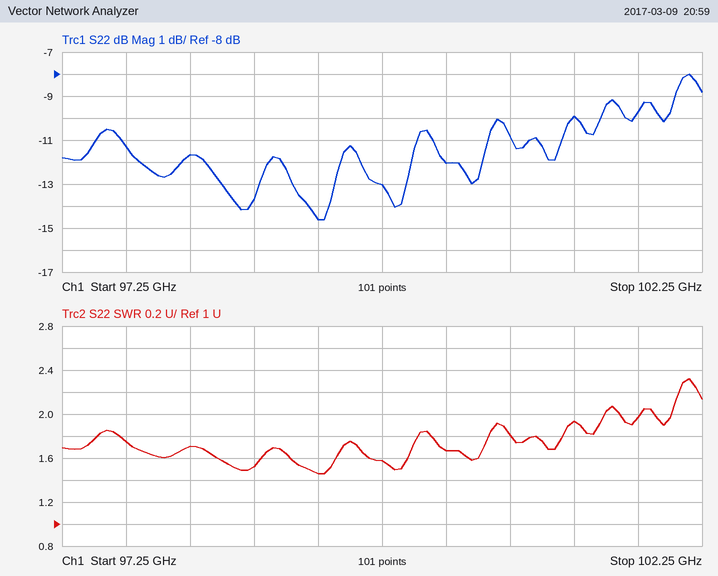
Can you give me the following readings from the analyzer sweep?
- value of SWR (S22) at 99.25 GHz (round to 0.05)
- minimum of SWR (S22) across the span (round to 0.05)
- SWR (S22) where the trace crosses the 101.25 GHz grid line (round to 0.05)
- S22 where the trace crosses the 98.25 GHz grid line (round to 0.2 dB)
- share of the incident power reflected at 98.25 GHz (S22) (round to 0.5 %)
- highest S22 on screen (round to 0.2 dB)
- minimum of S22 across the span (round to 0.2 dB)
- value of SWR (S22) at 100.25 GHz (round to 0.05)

1.45
1.45
1.95
-11.6 dB
7.0 %
-8.0 dB
-14.6 dB
1.65
